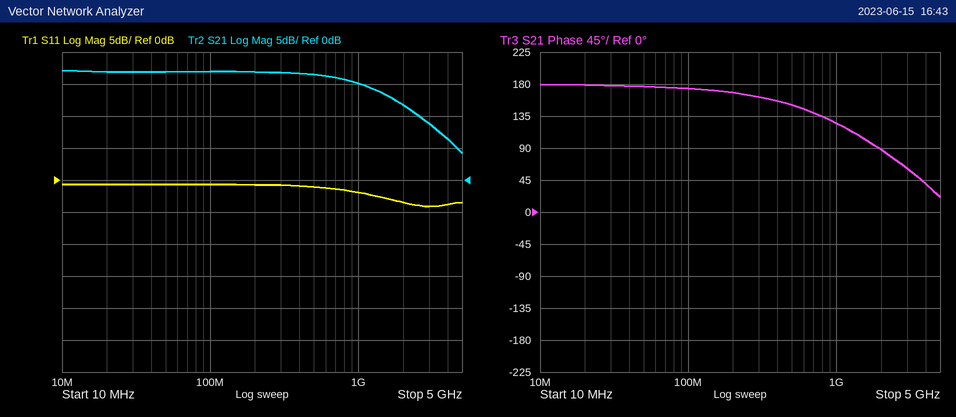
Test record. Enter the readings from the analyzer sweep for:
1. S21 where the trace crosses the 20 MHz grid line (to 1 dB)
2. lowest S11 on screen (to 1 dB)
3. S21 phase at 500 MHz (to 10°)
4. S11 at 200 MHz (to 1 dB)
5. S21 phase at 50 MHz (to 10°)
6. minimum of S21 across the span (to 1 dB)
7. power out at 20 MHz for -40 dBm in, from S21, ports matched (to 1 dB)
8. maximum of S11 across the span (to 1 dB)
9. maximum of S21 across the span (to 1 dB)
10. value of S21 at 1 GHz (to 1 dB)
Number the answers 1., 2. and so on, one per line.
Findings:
1. 17 dB
2. -4 dB
3. 150°
4. -1 dB
5. 180°
6. 4 dB
7. -23 dBm
8. -1 dB
9. 17 dB
10. 15 dB
